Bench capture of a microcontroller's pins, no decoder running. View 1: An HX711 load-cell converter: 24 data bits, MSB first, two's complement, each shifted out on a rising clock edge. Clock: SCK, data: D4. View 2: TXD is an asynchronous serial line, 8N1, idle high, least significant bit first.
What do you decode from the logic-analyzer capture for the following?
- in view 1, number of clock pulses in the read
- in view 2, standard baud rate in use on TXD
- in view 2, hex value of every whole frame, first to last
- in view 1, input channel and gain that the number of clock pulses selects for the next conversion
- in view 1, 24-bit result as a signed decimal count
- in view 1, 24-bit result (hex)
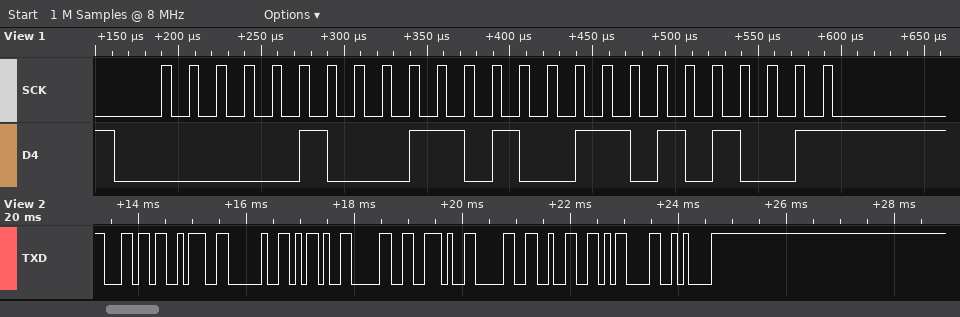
25
9600 baud
6C 3A 20 2D 30 2E 30 32 0D 0A
channel A, gain 128
289193
0x0469A9
